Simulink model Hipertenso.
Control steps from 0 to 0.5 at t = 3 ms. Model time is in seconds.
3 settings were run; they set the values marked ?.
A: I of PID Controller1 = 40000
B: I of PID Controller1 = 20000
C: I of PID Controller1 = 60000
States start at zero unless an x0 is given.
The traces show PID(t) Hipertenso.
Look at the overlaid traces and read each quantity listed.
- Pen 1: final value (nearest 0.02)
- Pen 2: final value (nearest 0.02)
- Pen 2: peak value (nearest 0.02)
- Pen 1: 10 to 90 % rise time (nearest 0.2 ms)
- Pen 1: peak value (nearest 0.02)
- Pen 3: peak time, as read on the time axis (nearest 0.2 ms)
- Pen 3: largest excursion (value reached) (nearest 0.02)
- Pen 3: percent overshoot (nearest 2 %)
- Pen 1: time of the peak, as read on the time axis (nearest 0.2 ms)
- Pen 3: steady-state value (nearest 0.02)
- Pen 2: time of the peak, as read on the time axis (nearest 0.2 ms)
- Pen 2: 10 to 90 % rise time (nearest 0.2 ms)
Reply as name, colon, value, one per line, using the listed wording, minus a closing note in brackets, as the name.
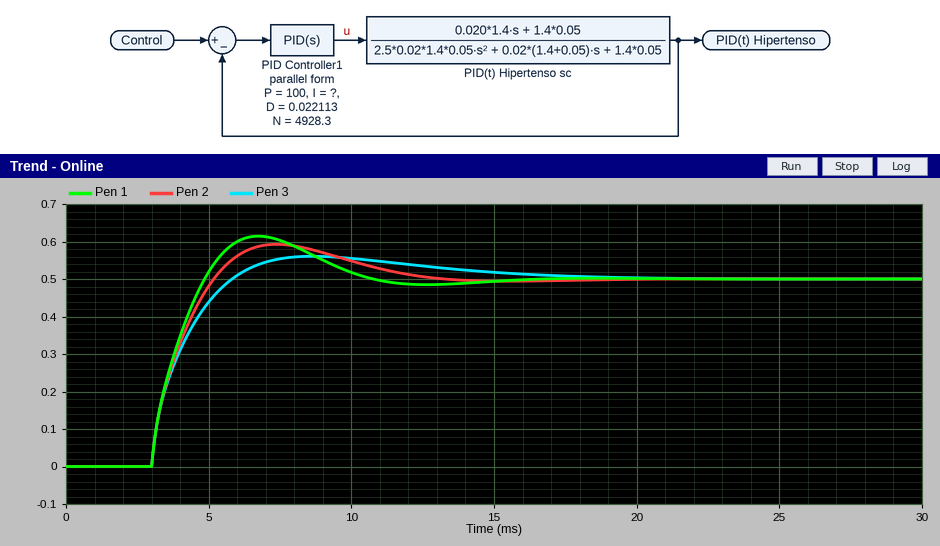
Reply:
Pen 1: final value: 0.50
Pen 2: final value: 0.50
Pen 2: peak value: 0.60
Pen 1: 10 to 90 % rise time: 1.4 ms
Pen 1: peak value: 0.62
Pen 3: peak time, as read on the time axis: 8.6 ms
Pen 3: largest excursion (value reached): 0.56
Pen 3: percent overshoot: 12 %
Pen 1: time of the peak, as read on the time axis: 6.8 ms
Pen 3: steady-state value: 0.50
Pen 2: time of the peak, as read on the time axis: 7.4 ms
Pen 2: 10 to 90 % rise time: 1.6 ms
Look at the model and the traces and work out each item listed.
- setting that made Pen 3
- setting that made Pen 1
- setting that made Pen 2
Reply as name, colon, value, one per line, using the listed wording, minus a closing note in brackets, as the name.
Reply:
setting that made Pen 3: B
setting that made Pen 1: C
setting that made Pen 2: A
